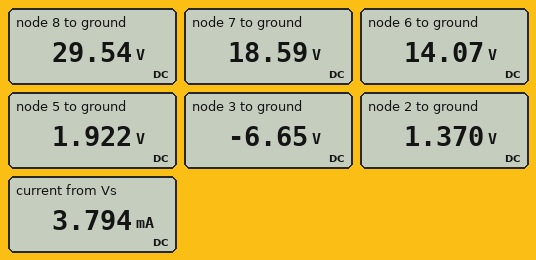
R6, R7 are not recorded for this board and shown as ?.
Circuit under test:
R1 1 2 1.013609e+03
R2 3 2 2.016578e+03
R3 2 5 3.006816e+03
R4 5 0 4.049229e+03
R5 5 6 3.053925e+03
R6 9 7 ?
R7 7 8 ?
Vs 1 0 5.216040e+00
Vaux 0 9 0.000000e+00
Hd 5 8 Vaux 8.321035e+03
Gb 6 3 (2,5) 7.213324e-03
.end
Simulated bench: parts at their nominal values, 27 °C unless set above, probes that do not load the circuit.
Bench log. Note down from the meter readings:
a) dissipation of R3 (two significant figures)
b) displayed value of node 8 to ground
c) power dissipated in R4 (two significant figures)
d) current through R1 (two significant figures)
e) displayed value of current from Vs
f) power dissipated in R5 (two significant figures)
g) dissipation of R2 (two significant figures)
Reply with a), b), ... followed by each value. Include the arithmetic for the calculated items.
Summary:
a) (1.922 V - 1.37 V)^2 / 3.007 kΩ = 100 µW
b) 29.54 V
c) (1.922 V)^2 / 4.049 kΩ = 910 µW
d) (5.216 V - 1.37 V) / 1.014 kΩ = 3.8 mA
e) 3.794 mA
f) (14.07 V - 1.922 V)^2 / 3.054 kΩ = 48 mW
g) (1.37 V - (-6.65 V))^2 / 2.017 kΩ = 32 mW
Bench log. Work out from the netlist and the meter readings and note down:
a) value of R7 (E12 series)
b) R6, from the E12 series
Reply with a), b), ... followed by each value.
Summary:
a) 3.3 kΩ
b) 5.6 kΩ
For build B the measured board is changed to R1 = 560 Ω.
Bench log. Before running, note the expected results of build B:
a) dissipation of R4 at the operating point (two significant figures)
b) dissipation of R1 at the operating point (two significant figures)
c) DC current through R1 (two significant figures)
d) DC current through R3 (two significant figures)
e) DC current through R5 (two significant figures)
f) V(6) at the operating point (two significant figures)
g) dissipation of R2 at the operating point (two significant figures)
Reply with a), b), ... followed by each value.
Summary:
a) 2.0 mW
b) 18 mW
c) 5.7 mA
d) 270 µA
e) 5.9 mA
f) 21 V
g) 71 mW
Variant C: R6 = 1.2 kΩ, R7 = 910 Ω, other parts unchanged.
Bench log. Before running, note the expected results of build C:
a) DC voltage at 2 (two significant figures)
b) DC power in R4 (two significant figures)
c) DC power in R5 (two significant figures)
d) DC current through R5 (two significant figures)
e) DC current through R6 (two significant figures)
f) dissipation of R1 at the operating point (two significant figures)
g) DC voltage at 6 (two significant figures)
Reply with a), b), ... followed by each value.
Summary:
a) 4.8 V
b) 5.8 mW
c) 580 µW
d) 440 µA
e) 780 µA
f) 180 µW
g) 6.2 V
